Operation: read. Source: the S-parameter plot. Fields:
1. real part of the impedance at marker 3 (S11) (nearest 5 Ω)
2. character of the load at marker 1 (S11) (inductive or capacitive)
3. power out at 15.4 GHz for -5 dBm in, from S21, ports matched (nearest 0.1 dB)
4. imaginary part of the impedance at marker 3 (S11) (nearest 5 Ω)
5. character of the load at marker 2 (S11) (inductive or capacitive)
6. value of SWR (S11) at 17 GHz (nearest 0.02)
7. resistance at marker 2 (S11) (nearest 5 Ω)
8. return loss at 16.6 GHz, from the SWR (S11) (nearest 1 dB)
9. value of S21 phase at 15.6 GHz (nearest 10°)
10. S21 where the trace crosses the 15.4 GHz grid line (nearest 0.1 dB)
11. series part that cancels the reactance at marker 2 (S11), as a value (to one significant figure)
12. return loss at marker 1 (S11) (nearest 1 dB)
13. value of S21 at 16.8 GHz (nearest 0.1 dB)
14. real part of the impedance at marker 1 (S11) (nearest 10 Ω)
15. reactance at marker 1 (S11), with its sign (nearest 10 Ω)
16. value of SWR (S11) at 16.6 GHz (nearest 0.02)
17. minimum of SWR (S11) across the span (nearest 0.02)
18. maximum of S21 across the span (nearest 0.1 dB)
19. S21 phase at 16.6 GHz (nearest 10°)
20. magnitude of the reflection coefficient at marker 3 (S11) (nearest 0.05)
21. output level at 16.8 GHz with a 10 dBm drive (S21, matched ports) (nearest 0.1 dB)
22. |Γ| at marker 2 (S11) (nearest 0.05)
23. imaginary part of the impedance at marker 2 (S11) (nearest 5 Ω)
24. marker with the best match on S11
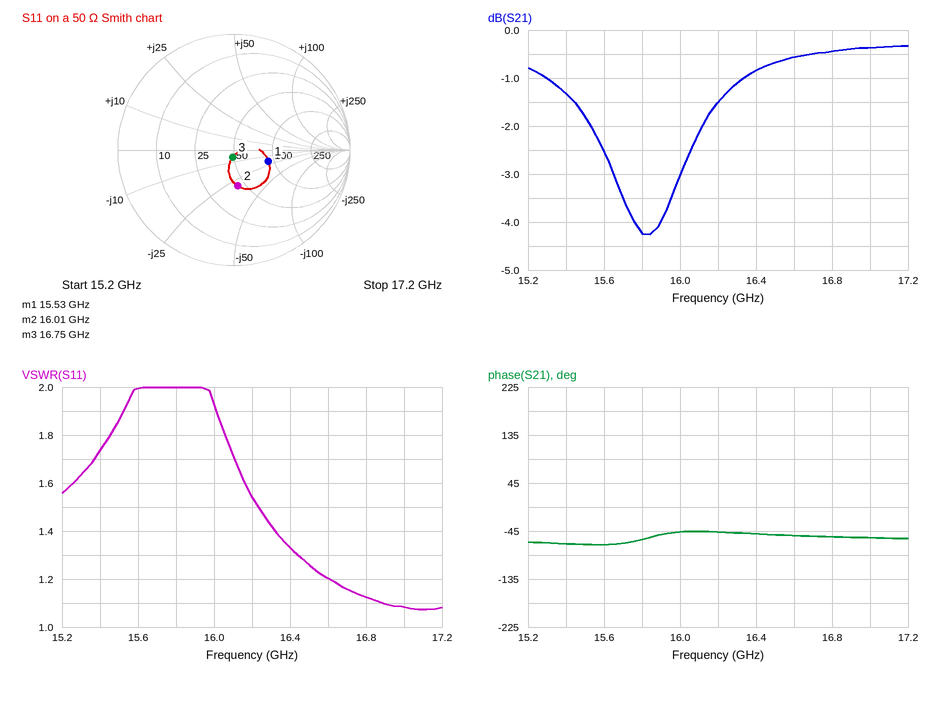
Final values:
50 Ω
capacitive
-6.3 dBm
-5 Ω
capacitive
1.08
45 Ω
21 dB
-70°
-1.3 dB
300 pH
10 dB
-0.4 dB
90 Ω
-20 Ω
1.20
1.08
-0.3 dB
-50°
0.05
9.6 dBm
0.30
-30 Ω
marker 3
